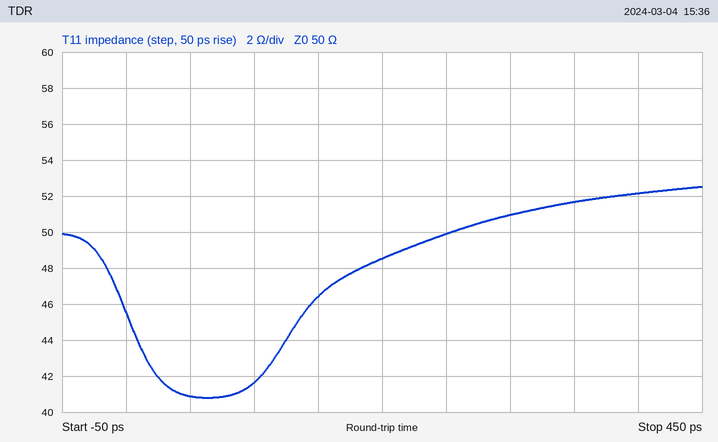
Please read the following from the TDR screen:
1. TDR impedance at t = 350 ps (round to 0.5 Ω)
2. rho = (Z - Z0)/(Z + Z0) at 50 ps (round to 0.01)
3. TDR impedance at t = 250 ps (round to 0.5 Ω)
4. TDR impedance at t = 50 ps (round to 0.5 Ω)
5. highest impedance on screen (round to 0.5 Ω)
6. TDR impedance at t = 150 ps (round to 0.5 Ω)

51.5 Ω
-0.10
50.0 Ω
41.0 Ω
52.5 Ω
46.5 Ω
